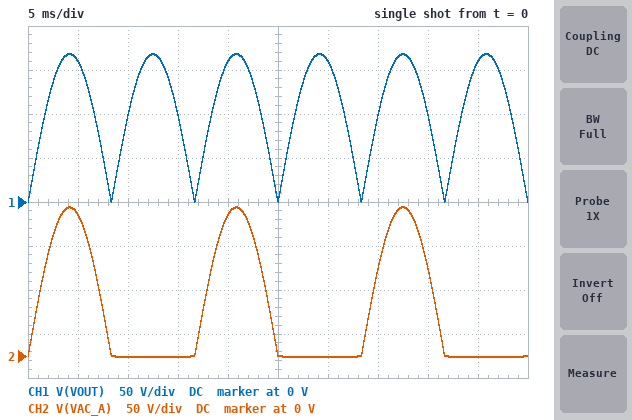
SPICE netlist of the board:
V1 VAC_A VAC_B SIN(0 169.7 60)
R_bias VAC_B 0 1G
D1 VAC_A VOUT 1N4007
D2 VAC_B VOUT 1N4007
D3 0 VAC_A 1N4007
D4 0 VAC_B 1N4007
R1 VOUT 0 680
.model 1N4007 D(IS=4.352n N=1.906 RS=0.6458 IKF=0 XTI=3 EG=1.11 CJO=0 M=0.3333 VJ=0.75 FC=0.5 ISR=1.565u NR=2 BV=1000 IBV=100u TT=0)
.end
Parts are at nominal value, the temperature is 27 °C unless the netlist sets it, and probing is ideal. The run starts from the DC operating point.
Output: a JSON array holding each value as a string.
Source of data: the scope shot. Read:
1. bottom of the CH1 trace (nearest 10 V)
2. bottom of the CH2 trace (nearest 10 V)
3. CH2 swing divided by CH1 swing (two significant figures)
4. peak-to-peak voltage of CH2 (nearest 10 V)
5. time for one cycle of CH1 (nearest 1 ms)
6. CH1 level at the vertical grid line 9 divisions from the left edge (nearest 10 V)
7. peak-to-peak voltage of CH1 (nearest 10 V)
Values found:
["0 V", "0 V", "1.0", "170 V", "8 ms", "160 V", "170 V"]
